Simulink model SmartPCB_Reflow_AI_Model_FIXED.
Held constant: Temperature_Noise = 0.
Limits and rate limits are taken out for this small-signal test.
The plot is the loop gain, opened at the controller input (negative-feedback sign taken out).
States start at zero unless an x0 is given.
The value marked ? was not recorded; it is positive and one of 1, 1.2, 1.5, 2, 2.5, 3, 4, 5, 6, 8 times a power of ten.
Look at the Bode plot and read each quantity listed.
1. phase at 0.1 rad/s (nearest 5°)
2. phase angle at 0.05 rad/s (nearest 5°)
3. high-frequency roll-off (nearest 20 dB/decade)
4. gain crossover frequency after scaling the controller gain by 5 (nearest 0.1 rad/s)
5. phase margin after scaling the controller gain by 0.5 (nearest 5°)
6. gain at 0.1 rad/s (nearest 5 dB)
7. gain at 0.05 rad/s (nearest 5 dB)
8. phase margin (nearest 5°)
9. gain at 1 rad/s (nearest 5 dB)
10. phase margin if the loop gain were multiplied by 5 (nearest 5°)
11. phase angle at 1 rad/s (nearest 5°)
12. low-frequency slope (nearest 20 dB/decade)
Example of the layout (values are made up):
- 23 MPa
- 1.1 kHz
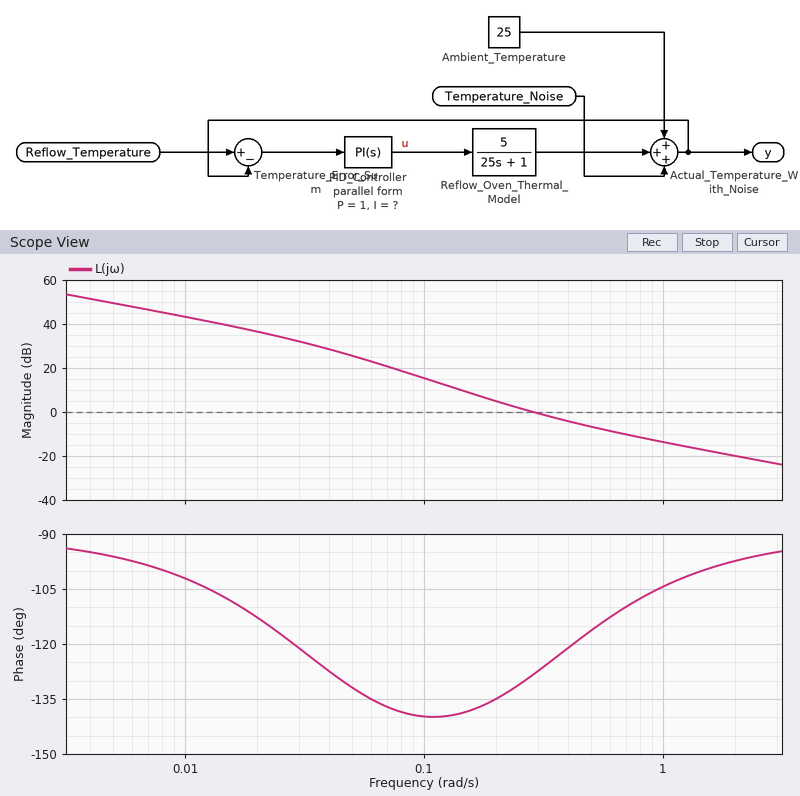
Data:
- -140°
- -130°
- -20 dB/decade
- 1.0 rad/s
- 45°
- 15 dB
- 25 dB
- 50°
- -15 dB
- 75°
- -105°
- -20 dB/decade
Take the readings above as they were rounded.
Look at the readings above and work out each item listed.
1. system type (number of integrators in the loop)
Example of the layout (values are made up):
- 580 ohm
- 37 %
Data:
- 1
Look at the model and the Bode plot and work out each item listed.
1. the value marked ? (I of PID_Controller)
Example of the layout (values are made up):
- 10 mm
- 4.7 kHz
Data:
- 0.3
